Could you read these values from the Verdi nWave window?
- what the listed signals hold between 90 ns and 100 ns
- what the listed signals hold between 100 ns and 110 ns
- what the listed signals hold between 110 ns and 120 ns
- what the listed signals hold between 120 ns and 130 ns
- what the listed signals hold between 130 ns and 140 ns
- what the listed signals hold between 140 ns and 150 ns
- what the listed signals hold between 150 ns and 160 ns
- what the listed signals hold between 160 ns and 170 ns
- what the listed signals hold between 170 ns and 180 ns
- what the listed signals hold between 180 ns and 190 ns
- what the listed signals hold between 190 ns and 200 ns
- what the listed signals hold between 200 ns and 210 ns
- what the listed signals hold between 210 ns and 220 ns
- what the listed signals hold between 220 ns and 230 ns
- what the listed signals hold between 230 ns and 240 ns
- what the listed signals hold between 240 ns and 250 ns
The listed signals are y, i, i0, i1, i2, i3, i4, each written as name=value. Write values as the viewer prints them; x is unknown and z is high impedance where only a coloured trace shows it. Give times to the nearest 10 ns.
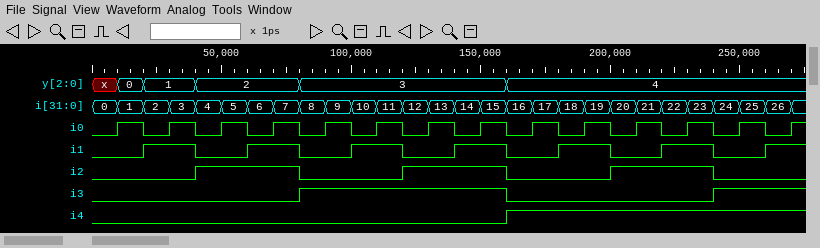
y=3, i=9, i0=1, i1=0, i2=0, i3=1, i4=0
y=3, i=10, i0=0, i1=1, i2=0, i3=1, i4=0
y=3, i=11, i0=1, i1=1, i2=0, i3=1, i4=0
y=3, i=12, i0=0, i1=0, i2=1, i3=1, i4=0
y=3, i=13, i0=1, i1=0, i2=1, i3=1, i4=0
y=3, i=14, i0=0, i1=1, i2=1, i3=1, i4=0
y=3, i=15, i0=1, i1=1, i2=1, i3=1, i4=0
y=4, i=16, i0=0, i1=0, i2=0, i3=0, i4=1
y=4, i=17, i0=1, i1=0, i2=0, i3=0, i4=1
y=4, i=18, i0=0, i1=1, i2=0, i3=0, i4=1
y=4, i=19, i0=1, i1=1, i2=0, i3=0, i4=1
y=4, i=20, i0=0, i1=0, i2=1, i3=0, i4=1
y=4, i=21, i0=1, i1=0, i2=1, i3=0, i4=1
y=4, i=22, i0=0, i1=1, i2=1, i3=0, i4=1
y=4, i=23, i0=1, i1=1, i2=1, i3=0, i4=1
y=4, i=24, i0=0, i1=0, i2=0, i3=1, i4=1
